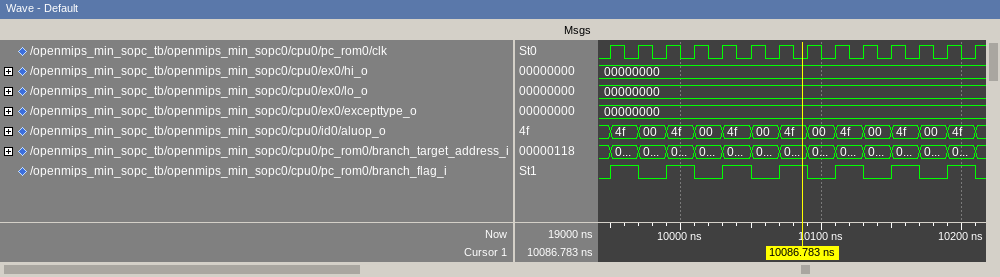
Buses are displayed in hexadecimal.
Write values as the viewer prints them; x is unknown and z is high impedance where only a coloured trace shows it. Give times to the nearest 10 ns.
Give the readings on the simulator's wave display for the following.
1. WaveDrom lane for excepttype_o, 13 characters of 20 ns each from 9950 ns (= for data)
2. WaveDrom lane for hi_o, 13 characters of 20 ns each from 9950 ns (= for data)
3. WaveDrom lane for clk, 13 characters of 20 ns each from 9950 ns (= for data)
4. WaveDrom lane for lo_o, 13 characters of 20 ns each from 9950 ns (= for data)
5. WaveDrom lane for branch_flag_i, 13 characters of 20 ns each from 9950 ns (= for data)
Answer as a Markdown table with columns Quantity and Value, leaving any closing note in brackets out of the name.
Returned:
| Quantity | Value |
|---|---|
| WaveDrom lane for excepttype_o, 13 characters of 20 ns each from 9950 ns | {name: 'excepttype_o', wave: '=............', data: '00000000'} |
| WaveDrom lane for hi_o, 13 characters of 20 ns each from 9950 ns | {name: 'hi_o', wave: '=............', data: '00000000'} |
| WaveDrom lane for clk, 13 characters of 20 ns each from 9950 ns | {name: 'clk', wave: 'p............'} |
| WaveDrom lane for lo_o, 13 characters of 20 ns each from 9950 ns | {name: 'lo_o', wave: '=............', data: '00000000'} |
| WaveDrom lane for branch_flag_i, 13 characters of 20 ns each from 9950 ns | {name: 'branch_flag_i', wave: '1010101010101'} |
